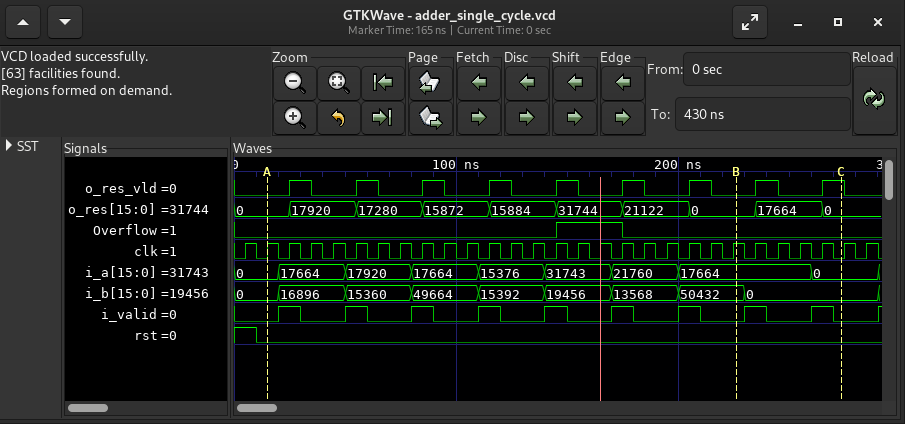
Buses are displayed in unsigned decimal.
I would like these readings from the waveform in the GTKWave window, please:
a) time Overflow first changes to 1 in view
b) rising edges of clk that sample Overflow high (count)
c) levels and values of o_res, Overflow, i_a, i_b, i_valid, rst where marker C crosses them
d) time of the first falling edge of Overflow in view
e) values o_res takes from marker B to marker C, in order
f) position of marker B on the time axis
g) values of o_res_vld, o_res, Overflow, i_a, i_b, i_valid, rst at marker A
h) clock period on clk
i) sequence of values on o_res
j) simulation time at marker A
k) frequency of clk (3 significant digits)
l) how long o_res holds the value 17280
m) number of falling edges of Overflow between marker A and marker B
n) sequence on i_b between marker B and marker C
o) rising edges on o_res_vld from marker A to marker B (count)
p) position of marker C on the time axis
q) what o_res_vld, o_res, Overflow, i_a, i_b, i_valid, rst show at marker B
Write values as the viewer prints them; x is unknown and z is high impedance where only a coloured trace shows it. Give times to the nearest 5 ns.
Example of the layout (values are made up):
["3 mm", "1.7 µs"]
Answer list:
["145 ns", "3", "o_res=0, Overflow=0, i_a=0, i_b=0, i_valid=0, rst=0", "175 ns", "0, 17664, 0", "225 ns", "o_res_vld=0, o_res=0, Overflow=0, i_a=0, i_b=0, i_valid=0, rst=0", "10 ns", "0, 17920, 17280, 15872, 15884, 31744, 21122, 0, 17664, 0", "15 ns", "100 MHz", "30 ns", "1", "50432, 0", "7", "275 ns", "o_res_vld=0, o_res=0, Overflow=0, i_a=17664, i_b=50432, i_valid=0, rst=0"]
